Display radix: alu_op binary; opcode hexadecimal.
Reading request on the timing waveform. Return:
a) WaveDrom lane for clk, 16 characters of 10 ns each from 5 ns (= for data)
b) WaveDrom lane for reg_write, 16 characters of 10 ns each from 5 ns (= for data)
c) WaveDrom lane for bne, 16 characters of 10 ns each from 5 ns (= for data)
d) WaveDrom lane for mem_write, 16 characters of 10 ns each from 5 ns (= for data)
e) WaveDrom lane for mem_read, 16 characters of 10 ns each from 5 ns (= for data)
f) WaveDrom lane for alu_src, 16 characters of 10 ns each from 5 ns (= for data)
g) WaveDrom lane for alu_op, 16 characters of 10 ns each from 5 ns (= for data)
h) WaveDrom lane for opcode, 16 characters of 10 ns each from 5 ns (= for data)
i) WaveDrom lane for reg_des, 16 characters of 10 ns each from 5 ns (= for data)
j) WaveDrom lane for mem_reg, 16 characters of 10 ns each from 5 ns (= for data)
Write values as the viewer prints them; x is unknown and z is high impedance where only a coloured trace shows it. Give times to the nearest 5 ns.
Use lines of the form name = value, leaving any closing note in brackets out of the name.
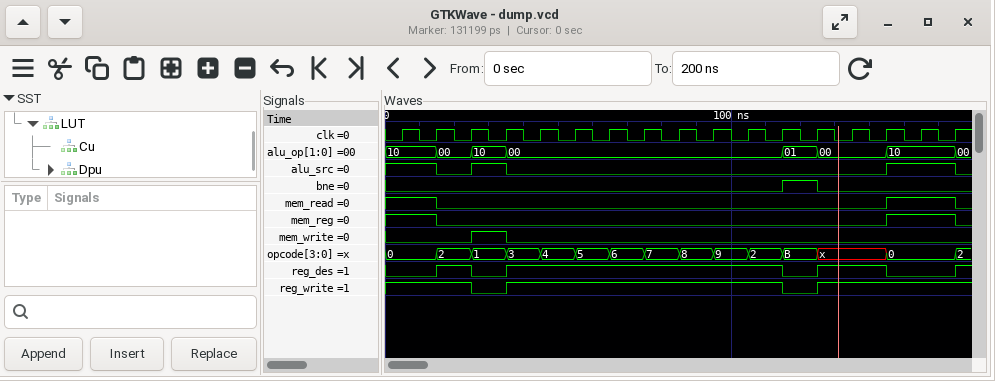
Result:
WaveDrom lane for clk, 16 characters of 10 ns each from 5 ns = {name: 'clk', wave: 'p...............'}
WaveDrom lane for reg_write, 16 characters of 10 ns each from 5 ns = {name: 'reg_write', wave: '1.01.......01...'}
WaveDrom lane for bne, 16 characters of 10 ns each from 5 ns = {name: 'bne', wave: '0..........10...'}
WaveDrom lane for mem_write, 16 characters of 10 ns each from 5 ns = {name: 'mem_write', wave: '0.10............'}
WaveDrom lane for mem_read, 16 characters of 10 ns each from 5 ns = {name: 'mem_read', wave: '10............1.'}
WaveDrom lane for alu_src, 16 characters of 10 ns each from 5 ns = {name: 'alu_src', wave: '1010..........1.'}
WaveDrom lane for alu_op, 16 characters of 10 ns each from 5 ns = {name: 'alu_op', wave: '====.......==.=.', data: '10 00 10 00 01 00 10'}
WaveDrom lane for opcode, 16 characters of 10 ns each from 5 ns = {name: 'opcode', wave: '============x.=.', data: '0 2 1 3 4 5 6 7 8 9 2 B 0'}
WaveDrom lane for reg_des, 16 characters of 10 ns each from 5 ns = {name: 'reg_des', wave: '0101.......01.0.'}
WaveDrom lane for mem_reg, 16 characters of 10 ns each from 5 ns = {name: 'mem_reg', wave: '10............1.'}
